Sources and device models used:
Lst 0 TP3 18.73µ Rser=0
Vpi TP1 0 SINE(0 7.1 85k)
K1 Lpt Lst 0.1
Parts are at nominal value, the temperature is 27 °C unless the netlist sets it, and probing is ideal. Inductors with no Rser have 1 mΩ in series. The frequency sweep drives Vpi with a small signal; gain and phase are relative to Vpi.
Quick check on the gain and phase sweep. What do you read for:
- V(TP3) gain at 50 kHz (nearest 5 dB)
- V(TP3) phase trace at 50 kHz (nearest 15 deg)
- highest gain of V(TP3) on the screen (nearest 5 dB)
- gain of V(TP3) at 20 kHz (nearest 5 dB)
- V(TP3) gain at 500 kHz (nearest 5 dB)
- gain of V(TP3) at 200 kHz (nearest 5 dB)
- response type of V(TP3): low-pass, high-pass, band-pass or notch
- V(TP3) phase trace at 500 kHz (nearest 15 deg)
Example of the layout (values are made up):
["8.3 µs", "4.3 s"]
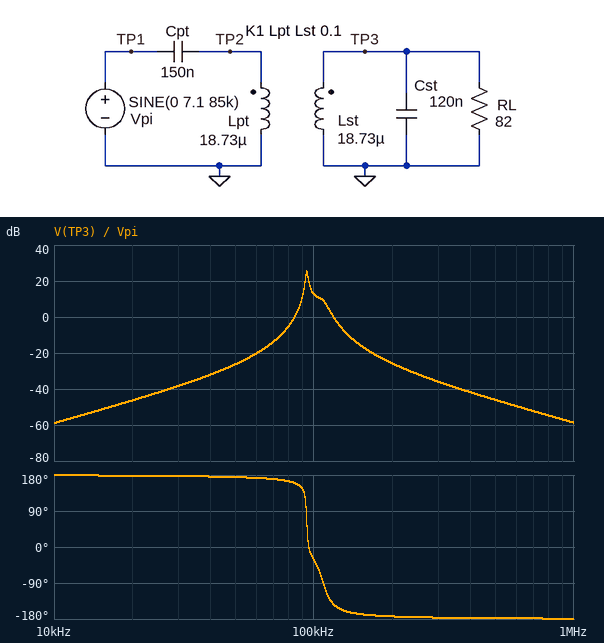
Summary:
["-25 dB", "180 deg", "25 dB", "-45 dB", "-45 dB", "-25 dB", "band-pass", "-180 deg"]
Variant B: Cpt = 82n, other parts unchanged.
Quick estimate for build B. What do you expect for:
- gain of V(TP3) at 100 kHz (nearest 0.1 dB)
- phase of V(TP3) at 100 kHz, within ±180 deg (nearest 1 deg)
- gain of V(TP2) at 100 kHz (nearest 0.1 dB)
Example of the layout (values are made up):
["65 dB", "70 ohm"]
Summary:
["-1.2 dB", "124 deg", "4.3 dB"]
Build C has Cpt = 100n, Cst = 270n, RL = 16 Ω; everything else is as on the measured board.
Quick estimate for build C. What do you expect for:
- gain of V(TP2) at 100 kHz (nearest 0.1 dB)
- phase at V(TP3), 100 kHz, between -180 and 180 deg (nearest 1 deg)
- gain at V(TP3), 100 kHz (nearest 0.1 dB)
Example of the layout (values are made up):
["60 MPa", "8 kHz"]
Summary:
["8.5 dB", "36 deg", "-13.2 dB"]
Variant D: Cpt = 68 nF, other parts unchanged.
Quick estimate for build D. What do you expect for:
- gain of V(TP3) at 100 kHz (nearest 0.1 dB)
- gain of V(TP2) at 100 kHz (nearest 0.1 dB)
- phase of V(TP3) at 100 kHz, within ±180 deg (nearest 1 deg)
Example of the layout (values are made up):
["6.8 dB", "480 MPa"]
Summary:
["-4.9 dB", "0.5 dB", "126 deg"]
